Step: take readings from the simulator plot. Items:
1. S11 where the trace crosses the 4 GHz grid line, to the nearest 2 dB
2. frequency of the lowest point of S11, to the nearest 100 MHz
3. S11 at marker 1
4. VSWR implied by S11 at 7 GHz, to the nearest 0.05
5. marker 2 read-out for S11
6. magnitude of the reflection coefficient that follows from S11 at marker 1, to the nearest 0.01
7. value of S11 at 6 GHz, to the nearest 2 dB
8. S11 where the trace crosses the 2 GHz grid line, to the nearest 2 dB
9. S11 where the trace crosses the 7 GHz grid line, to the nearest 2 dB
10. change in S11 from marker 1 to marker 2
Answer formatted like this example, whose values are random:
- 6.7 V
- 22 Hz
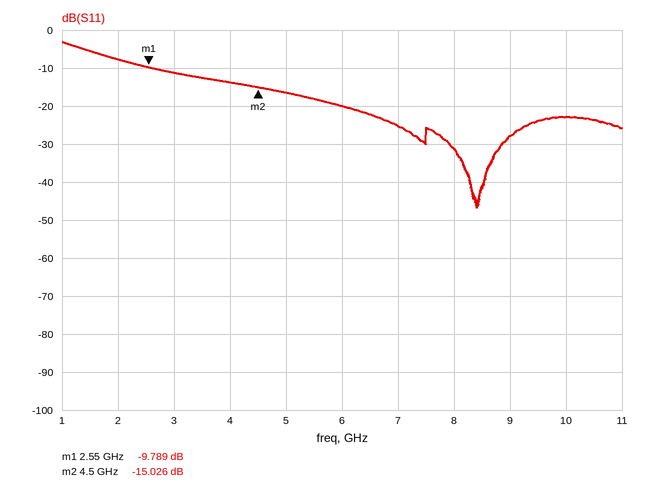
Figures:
- -14 dB
- 8.4 GHz
- -9.789 dB
- 1.10
- -15.026 dB
- 0.32
- -20 dB
- -8 dB
- -26 dB
- -5.237 dB
